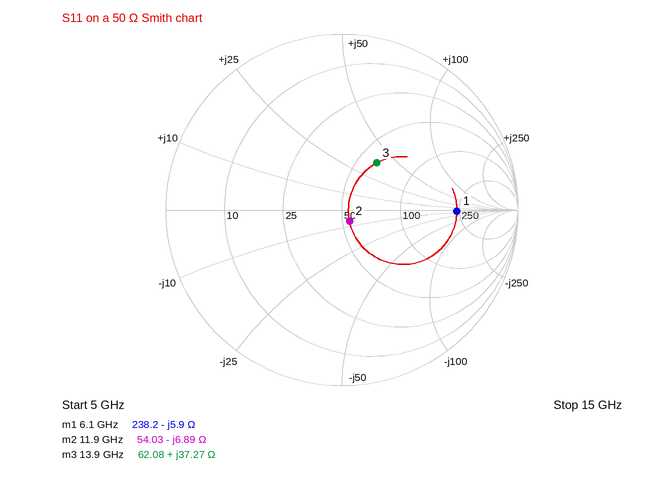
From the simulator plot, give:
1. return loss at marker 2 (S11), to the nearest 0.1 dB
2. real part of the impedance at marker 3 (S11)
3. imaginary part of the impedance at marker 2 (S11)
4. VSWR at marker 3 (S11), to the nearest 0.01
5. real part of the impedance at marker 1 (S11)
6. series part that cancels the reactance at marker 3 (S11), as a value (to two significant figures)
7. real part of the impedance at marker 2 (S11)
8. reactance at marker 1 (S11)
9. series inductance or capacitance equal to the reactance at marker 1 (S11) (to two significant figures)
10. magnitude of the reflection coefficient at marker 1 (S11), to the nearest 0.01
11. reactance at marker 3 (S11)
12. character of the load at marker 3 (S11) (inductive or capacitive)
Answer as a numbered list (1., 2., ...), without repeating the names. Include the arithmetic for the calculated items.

1. 22.3 dB
2. 62.08 Ω
3. -6.89 Ω
4. 1.99
5. 238.2 Ω
6. C = 1/(2π × 13.9 GHz × 37.27 Ω) ≈ 307 fF, so 310 fF to two significant figures
7. 54.03 Ω
8. -5.9 Ω
9. C = 1/(2π × 6.1 GHz × 5.9 Ω) ≈ 4.4 pF
10. 0.65
11. +37.27 Ω
12. inductive
